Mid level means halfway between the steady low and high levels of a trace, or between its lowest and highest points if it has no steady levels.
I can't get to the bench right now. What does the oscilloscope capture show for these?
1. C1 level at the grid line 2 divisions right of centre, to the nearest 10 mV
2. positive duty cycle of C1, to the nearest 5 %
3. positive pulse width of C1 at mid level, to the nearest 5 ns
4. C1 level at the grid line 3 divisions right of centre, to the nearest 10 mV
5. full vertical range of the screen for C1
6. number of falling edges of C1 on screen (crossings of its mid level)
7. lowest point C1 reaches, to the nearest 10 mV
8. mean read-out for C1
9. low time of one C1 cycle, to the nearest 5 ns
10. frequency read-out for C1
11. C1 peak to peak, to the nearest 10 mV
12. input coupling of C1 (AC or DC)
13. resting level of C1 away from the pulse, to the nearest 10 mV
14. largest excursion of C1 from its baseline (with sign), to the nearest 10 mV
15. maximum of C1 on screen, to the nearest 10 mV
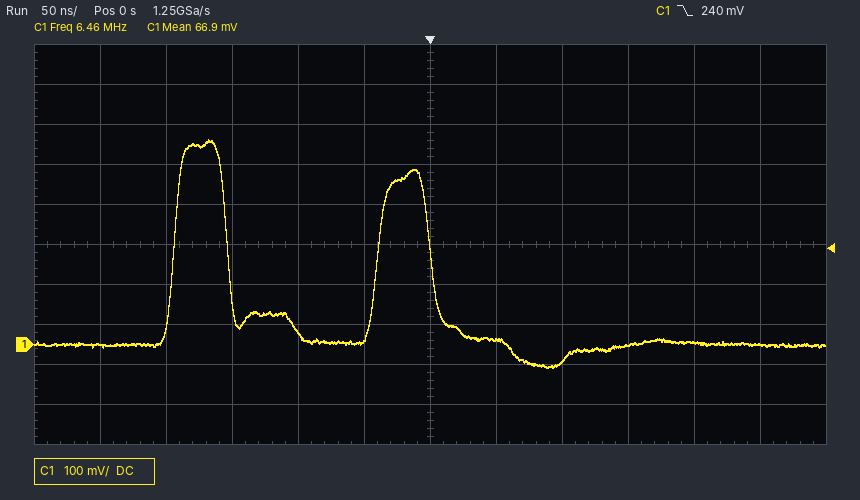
-40 mV
25 %
40 ns
0 mV
1 V
2
-60 mV
66.9 mV
115 ns
6.46 MHz
570 mV
DC
0 mV
+510 mV
510 mV
